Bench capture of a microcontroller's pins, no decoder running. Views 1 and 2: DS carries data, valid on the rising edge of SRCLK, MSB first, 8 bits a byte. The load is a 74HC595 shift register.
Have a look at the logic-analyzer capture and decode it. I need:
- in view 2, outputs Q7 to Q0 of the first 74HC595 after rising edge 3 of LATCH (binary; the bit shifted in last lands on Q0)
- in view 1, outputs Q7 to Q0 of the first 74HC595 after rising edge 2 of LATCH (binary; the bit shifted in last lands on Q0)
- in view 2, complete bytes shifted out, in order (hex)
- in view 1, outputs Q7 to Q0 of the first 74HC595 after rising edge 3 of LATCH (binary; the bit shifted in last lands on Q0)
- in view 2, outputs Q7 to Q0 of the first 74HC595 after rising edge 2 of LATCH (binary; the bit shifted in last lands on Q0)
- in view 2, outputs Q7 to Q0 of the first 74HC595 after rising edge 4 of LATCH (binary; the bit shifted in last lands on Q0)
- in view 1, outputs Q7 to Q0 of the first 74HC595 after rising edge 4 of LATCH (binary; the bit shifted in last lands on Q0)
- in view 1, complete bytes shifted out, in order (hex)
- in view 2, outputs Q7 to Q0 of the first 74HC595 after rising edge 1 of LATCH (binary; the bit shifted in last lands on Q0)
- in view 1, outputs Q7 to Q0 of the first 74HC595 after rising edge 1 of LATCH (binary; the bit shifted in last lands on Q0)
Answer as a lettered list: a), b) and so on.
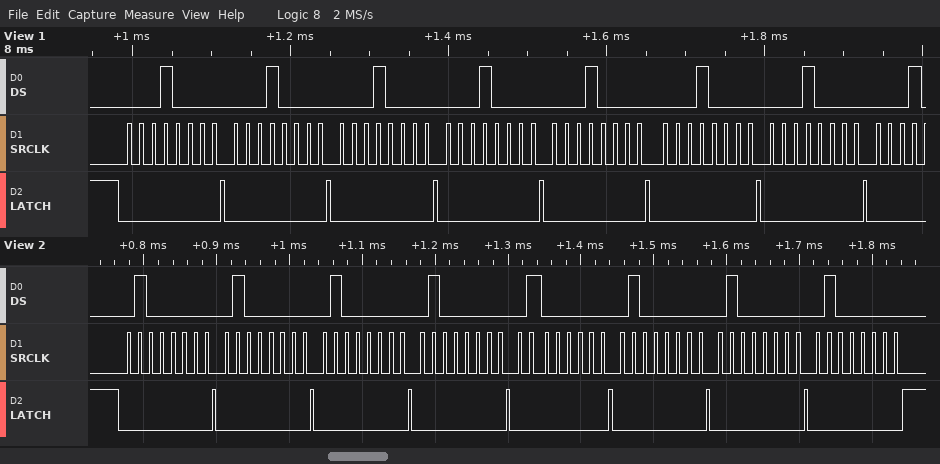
a) 01000000
b) 00010000
c) 40 40 40 40 40 40 40 40
d) 00010000
e) 01000000
f) 01000000
g) 00010000
h) 0x10 0x10 0x10 0x10 0x10 0x10 0x10
i) 01000000
j) 00010000
